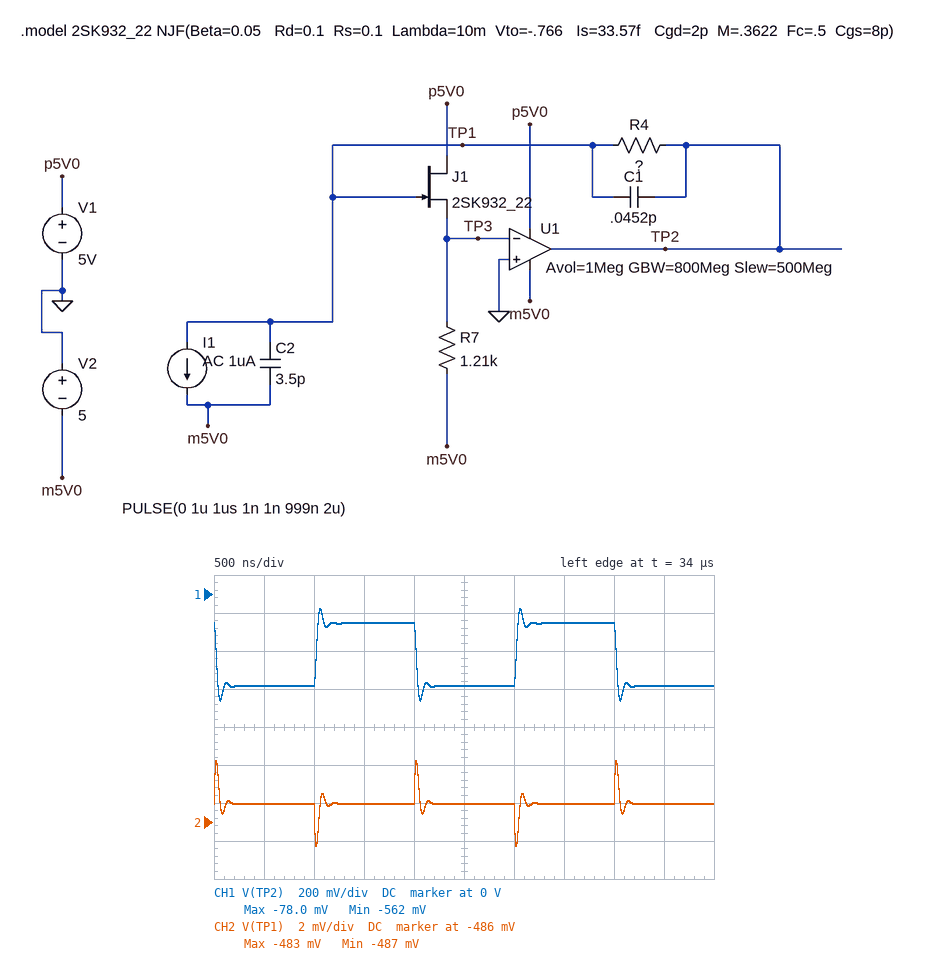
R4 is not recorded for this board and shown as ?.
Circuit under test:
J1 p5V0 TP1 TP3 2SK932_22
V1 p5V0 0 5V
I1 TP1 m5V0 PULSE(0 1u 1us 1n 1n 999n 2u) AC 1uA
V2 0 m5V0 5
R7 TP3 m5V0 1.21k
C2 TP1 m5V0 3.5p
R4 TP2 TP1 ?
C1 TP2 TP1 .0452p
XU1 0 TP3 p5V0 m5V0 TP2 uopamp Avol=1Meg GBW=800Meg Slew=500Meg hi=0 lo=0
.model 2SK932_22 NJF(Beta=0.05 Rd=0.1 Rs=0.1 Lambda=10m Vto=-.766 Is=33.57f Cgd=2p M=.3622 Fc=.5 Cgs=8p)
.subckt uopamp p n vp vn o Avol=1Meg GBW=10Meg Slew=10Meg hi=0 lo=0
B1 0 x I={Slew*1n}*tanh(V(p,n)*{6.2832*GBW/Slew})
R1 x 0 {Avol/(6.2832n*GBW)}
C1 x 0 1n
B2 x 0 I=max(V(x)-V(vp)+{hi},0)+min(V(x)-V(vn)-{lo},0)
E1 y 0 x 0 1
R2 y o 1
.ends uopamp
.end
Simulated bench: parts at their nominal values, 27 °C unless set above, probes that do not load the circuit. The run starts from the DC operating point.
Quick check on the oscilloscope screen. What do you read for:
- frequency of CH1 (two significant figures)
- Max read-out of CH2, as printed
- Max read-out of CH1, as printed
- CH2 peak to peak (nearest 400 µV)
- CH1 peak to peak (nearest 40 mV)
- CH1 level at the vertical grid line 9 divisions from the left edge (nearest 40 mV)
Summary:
500 kHz
-483 mV
-78.0 mV
4.4 mV
480 mV
-480 mV
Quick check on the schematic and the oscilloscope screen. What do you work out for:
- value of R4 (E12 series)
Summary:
330 kΩ
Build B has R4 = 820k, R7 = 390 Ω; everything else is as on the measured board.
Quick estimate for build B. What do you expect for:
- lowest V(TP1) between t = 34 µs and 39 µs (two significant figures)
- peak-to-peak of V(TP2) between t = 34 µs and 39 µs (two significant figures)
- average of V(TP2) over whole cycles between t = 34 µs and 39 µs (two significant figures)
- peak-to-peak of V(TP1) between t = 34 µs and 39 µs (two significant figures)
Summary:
-270 mV
930 mV
140 mV
5.8 mV
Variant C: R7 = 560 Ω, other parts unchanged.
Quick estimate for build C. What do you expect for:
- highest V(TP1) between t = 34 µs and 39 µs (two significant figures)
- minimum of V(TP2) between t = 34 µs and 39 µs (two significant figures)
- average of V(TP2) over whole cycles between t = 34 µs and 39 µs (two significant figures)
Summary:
-350 mV
-430 mV
-190 mV
